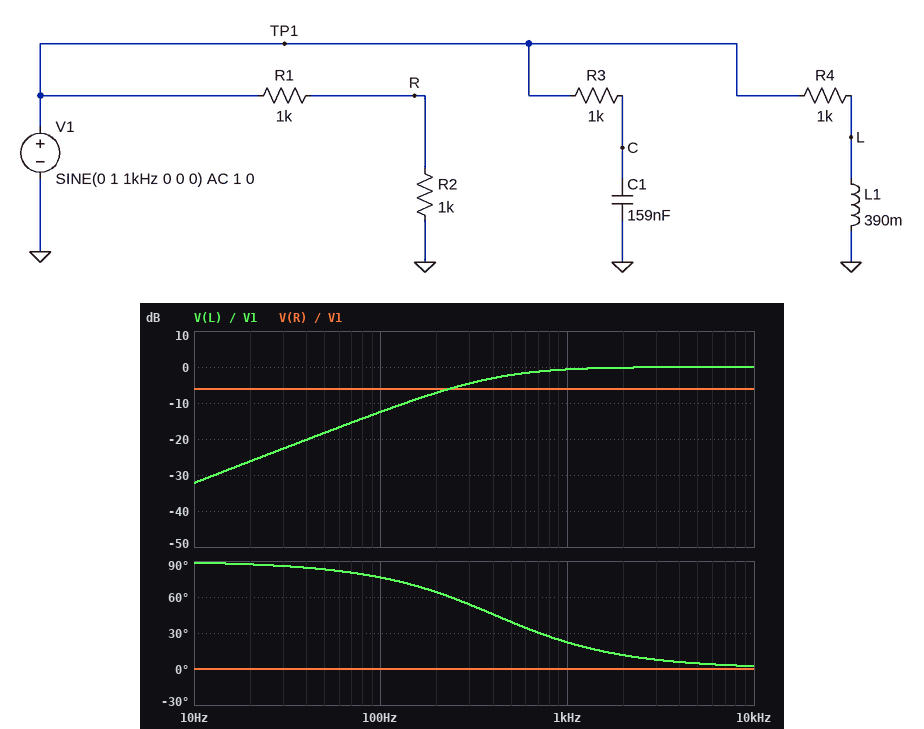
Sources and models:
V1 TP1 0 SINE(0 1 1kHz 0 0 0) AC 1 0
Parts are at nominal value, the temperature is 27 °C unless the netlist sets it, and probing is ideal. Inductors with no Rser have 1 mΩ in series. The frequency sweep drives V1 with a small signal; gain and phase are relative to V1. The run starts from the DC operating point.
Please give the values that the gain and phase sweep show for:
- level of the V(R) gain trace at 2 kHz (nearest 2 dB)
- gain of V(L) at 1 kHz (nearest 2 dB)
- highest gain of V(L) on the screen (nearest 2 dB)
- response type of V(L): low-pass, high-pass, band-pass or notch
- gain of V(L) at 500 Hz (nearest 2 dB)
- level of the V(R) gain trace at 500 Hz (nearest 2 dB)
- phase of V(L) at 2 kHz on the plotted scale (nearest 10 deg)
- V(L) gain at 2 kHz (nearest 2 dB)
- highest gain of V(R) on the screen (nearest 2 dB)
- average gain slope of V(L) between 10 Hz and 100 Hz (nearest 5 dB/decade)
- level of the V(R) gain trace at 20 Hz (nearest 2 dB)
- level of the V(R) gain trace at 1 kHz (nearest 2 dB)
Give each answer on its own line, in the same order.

-6 dB
0 dB
0 dB
high-pass
-2 dB
-6 dB
10 deg
0 dB
-6 dB
20 dB/decade
-6 dB
-6 dB
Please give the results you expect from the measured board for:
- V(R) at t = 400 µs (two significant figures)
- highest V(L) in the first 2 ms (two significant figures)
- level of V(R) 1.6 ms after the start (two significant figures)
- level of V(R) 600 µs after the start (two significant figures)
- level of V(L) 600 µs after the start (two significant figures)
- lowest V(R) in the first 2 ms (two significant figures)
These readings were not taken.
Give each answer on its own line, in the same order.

290 mV
910 mV
-290 mV
-290 mV
-860 mV
-500 mV
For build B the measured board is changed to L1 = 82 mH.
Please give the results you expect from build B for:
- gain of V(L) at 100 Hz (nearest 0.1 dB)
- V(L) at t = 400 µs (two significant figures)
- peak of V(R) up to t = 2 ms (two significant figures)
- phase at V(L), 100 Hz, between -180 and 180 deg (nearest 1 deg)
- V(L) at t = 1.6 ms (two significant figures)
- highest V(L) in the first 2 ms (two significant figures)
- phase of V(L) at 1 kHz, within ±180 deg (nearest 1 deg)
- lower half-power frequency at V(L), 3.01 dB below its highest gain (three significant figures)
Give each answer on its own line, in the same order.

-25.8 dB
-210 mV
500 mV
87 deg
-450 mV
460 mV
63 deg
1.94 kHz
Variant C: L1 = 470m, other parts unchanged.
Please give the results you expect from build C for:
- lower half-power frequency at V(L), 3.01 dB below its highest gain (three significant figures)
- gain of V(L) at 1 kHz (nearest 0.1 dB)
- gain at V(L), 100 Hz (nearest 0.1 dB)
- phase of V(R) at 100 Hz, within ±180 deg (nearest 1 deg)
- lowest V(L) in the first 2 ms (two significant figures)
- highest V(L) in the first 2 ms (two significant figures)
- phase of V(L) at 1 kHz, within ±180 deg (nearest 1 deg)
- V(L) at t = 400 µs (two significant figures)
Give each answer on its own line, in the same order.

339 Hz
-0.5 dB
-11.0 dB
0 deg
-1.0 V
920 mV
19 deg
150 mV
